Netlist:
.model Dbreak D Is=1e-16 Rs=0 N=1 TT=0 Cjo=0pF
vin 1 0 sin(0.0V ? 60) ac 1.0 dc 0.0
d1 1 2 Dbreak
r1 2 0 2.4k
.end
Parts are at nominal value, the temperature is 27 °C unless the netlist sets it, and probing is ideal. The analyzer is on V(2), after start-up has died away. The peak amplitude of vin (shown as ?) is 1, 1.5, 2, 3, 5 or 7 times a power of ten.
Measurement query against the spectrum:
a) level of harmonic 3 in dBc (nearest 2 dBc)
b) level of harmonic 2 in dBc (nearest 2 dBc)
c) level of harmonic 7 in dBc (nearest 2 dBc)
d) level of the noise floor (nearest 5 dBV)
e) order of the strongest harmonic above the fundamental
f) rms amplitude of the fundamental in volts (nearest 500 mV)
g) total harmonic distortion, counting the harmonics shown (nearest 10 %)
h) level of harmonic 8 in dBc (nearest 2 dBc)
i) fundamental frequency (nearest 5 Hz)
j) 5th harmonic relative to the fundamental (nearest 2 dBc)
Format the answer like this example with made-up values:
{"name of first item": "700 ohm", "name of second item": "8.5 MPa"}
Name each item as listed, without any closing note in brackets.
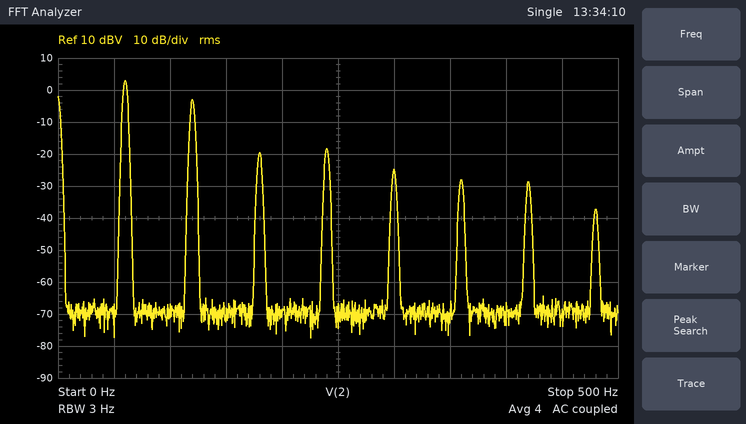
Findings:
{"level of harmonic 3 in dBc": "-22 dBc", "level of harmonic 2 in dBc": "-6 dBc", "level of harmonic 7 in dBc": "-32 dBc", "level of the noise floor": "-70 dBV", "order of the strongest harmonic above the fundamental": "2", "rms amplitude of the fundamental in volts": "1.5 V", "total harmonic distortion, counting the harmonics shown": "50 %", "level of harmonic 8 in dBc": "-40 dBc", "fundamental frequency": "60 Hz", "5th harmonic relative to the fundamental": "-28 dBc"}
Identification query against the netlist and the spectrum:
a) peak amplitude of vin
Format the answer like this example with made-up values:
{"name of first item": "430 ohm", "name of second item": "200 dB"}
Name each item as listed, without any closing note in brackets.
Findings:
{"peak amplitude of vin": "5 V"}
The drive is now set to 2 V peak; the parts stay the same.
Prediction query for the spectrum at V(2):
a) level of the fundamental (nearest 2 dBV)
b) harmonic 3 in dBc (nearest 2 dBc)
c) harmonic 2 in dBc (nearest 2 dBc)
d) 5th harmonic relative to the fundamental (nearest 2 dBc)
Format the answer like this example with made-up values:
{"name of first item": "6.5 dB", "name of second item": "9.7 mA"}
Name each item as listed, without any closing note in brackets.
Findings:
{"level of the fundamental": "-8 dBV", "harmonic 3 in dBc": "-14 dBc", "harmonic 2 in dBc": "-4 dBc", "5th harmonic relative to the fundamental": "-22 dBc"}
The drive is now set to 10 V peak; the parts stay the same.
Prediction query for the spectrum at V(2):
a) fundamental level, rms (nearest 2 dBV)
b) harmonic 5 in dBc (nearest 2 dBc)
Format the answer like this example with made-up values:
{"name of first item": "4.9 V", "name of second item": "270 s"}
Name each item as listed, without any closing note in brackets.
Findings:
{"fundamental level, rms": "10 dBV", "harmonic 5 in dBc": "-34 dBc"}
